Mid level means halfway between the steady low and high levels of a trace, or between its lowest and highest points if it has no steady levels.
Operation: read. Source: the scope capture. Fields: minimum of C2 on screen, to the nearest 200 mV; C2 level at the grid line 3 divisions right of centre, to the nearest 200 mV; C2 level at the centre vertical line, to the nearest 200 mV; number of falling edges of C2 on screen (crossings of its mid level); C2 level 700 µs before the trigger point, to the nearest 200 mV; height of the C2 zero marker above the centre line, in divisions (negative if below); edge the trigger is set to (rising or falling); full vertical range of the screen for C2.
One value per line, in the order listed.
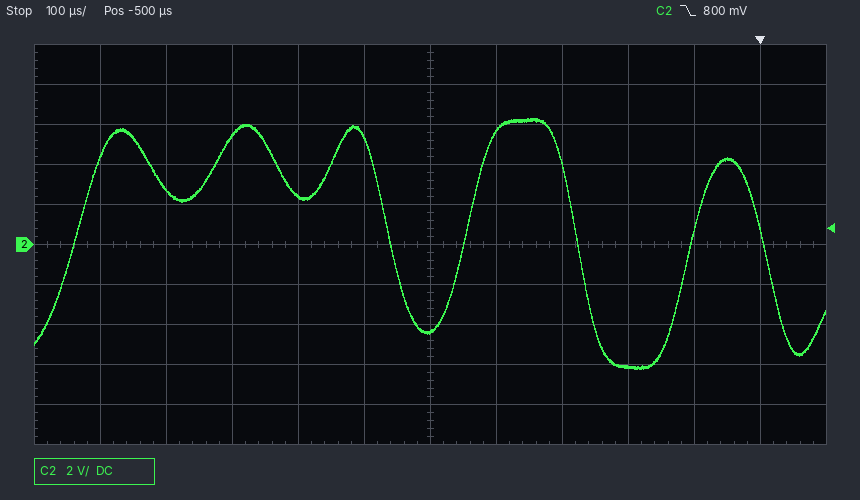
-6.2 V
-6.2 V
-4.4 V
3
2.4 V
0.0 div
falling
20 V
